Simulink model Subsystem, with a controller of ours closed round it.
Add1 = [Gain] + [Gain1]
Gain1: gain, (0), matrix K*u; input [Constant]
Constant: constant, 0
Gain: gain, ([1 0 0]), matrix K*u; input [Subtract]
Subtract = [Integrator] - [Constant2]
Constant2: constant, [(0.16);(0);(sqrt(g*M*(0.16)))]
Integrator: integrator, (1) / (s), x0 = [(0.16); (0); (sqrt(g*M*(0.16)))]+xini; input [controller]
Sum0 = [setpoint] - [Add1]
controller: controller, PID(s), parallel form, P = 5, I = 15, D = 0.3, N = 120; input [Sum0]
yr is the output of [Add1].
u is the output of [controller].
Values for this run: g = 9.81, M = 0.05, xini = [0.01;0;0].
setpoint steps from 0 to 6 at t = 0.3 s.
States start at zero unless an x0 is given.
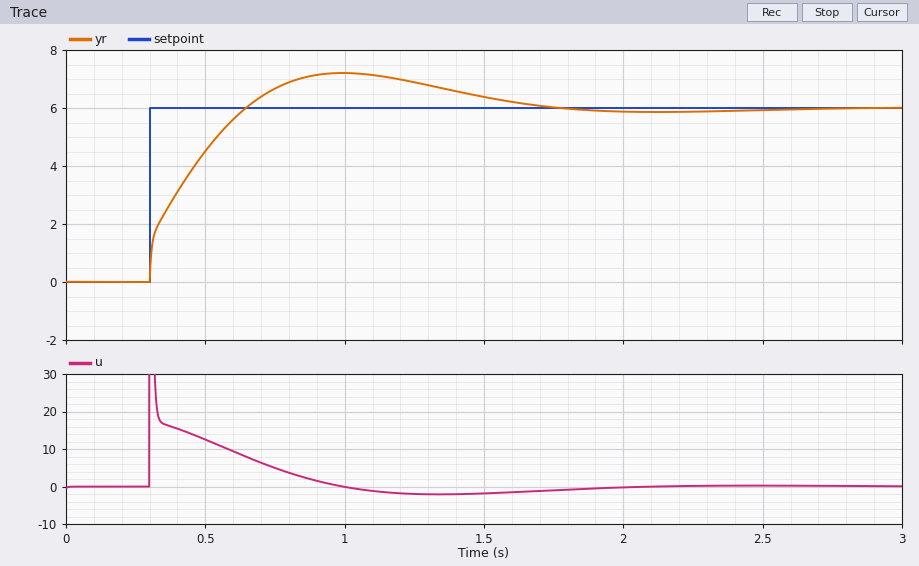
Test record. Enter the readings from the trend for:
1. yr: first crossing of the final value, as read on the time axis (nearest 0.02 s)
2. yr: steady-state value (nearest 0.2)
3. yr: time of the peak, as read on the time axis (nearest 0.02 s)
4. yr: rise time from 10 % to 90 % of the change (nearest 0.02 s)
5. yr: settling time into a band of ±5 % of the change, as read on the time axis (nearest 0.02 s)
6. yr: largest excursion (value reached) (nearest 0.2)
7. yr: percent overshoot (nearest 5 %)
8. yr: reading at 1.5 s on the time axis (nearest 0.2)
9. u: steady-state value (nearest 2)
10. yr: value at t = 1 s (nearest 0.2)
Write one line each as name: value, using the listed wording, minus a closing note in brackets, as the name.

yr: first crossing of the final value, as read on the time axis: 0.64 s
yr: steady-state value: 6.0
yr: time of the peak, as read on the time axis: 1.00 s
yr: rise time from 10 % to 90 % of the change: 0.28 s
yr: settling time into a band of ±5 % of the change, as read on the time axis: 1.54 s
yr: largest excursion (value reached): 7.2
yr: percent overshoot: 20 %
yr: reading at 1.5 s on the time axis: 6.4
u: steady-state value: 0
yr: value at t = 1 s: 7.2
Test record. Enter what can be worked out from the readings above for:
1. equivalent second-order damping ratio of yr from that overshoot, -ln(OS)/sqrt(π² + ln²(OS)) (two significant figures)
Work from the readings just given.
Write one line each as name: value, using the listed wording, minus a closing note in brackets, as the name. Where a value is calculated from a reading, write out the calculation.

equivalent second-order damping ratio of yr from that overshoot, -ln(OS)/sqrt(π² + ln²(OS)): ln(0.2) = -1.609; 1.609 / sqrt(9.870 + 2.590) = 0.46
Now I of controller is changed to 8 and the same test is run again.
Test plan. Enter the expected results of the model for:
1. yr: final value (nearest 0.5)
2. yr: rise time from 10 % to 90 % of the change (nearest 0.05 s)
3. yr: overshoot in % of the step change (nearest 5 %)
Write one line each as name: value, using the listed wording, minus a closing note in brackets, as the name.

yr: final value: 6.0
yr: rise time from 10 % to 90 % of the change: 0.35 s
yr: overshoot in % of the step change: 15 %
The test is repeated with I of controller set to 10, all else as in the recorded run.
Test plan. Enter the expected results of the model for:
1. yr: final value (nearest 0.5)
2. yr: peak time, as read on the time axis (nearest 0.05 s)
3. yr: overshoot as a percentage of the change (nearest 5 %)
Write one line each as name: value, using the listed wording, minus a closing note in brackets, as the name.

yr: final value: 6.0
yr: peak time, as read on the time axis: 1.10 s
yr: overshoot as a percentage of the change: 15 %
